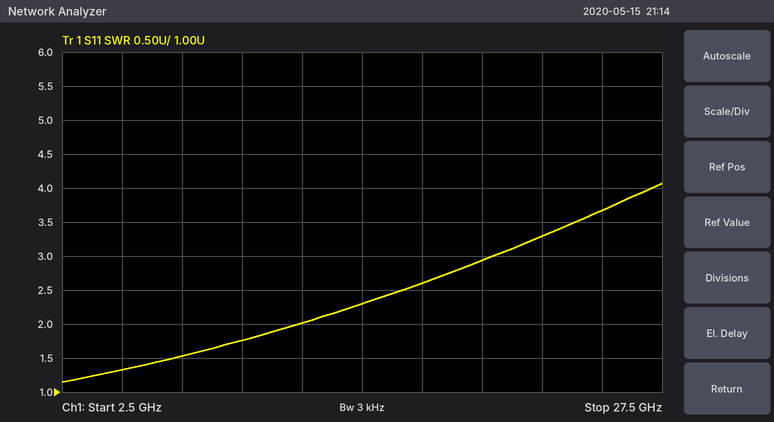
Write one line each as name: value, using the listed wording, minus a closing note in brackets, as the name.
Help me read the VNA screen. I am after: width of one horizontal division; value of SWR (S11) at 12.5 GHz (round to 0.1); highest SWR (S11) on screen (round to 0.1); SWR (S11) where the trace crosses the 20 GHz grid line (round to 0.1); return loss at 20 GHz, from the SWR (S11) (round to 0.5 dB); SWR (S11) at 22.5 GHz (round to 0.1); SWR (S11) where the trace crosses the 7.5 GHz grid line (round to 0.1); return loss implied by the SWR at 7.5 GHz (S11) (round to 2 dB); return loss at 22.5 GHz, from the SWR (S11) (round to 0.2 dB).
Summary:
width of one horizontal division: 2.5 GHz
value of SWR (S11) at 12.5 GHz: 2.0
highest SWR (S11) on screen: 4.1
SWR (S11) where the trace crosses the 20 GHz grid line: 2.9
return loss at 20 GHz, from the SWR (S11): 6.0 dB
SWR (S11) at 22.5 GHz: 3.3
SWR (S11) where the trace crosses the 7.5 GHz grid line: 1.5
return loss implied by the SWR at 7.5 GHz (S11): 14 dB
return loss at 22.5 GHz, from the SWR (S11): 5.4 dB
